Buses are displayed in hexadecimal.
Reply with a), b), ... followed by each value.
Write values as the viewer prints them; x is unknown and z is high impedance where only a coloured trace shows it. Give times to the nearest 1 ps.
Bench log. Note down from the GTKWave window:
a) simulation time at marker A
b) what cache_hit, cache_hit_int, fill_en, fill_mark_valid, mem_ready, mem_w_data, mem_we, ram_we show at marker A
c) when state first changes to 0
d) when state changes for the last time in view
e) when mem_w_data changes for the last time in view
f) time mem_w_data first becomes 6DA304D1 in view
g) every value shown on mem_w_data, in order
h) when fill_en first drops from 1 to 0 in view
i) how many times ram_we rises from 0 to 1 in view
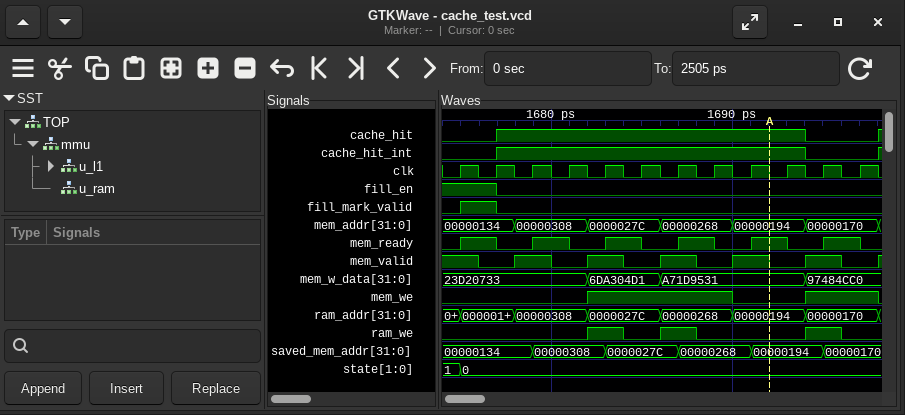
a) 1692 ps
b) cache_hit=1, cache_hit_int=1, fill_en=0, fill_mark_valid=0, mem_ready=1, mem_w_data=A71D9531, mem_we=0, ram_we=0
c) 1675 ps
d) 1675 ps
e) 1694 ps
f) 1682 ps
g) 23D20733, 6DA304D1, A71D9531, 97484CC0
h) 1677 ps
i) 3
